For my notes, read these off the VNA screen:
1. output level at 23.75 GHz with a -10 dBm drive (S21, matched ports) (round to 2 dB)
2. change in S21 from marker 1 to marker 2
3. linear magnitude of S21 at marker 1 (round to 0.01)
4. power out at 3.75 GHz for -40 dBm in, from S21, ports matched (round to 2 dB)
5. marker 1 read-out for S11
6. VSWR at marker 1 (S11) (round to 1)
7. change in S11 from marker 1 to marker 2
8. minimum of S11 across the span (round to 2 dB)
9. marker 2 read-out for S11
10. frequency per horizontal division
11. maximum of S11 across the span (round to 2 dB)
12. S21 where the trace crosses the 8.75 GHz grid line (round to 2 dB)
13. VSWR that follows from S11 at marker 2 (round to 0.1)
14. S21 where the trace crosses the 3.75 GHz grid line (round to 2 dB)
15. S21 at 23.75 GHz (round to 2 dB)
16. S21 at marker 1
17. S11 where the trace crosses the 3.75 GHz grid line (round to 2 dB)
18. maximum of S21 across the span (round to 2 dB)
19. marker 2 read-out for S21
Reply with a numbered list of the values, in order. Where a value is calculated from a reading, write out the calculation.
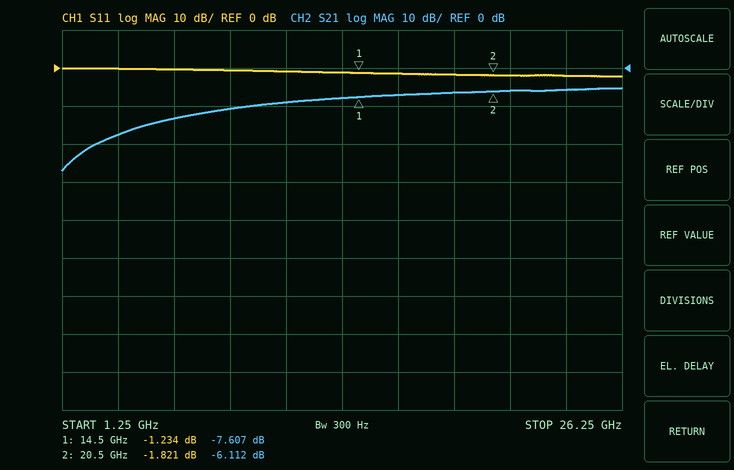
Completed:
1. -10 dBm + (-6 dB) = -16 dBm
2. -6.112 − (-7.607) = 1.495 dB
3. 10^(-7.607/20) ≈ 0.42
4. -40 dBm + (-18 dB) = -58 dBm
5. -1.234 dB
6. (1 + 0.8676)/(1 − 0.8676) ≈ 14
7. -1.821 − (-1.234) = -0.587 dB
8. -2 dB
9. -1.821 dB
10. 2.5 GHz
11. 0 dB
12. -10 dB
13. (1 + 0.8109)/(1 − 0.8109) ≈ 9.6
14. -18 dB
15. -6 dB
16. -7.607 dB
17. 0 dB
18. -6 dB
19. -6.112 dB
